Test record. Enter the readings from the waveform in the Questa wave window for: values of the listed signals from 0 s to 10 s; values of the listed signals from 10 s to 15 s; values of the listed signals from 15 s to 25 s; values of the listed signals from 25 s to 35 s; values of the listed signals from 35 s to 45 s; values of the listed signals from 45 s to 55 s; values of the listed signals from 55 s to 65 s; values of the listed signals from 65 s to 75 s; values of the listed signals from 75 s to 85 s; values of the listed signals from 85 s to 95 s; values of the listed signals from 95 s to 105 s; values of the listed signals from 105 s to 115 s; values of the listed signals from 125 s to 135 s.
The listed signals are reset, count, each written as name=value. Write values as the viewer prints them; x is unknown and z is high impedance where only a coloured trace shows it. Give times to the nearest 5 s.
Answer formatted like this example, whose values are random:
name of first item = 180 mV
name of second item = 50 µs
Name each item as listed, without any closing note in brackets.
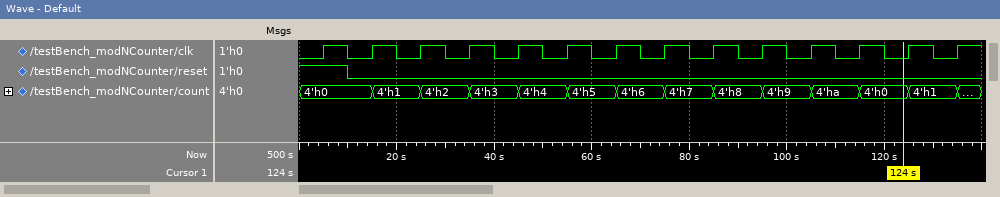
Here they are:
values of the listed signals from 0 s to 10 s = reset=1, count=4'h0
values of the listed signals from 10 s to 15 s = reset=0, count=4'h0
values of the listed signals from 15 s to 25 s = reset=0, count=4'h1
values of the listed signals from 25 s to 35 s = reset=0, count=4'h2
values of the listed signals from 35 s to 45 s = reset=0, count=4'h3
values of the listed signals from 45 s to 55 s = reset=0, count=4'h4
values of the listed signals from 55 s to 65 s = reset=0, count=4'h5
values of the listed signals from 65 s to 75 s = reset=0, count=4'h6
values of the listed signals from 75 s to 85 s = reset=0, count=4'h7
values of the listed signals from 85 s to 95 s = reset=0, count=4'h8
values of the listed signals from 95 s to 105 s = reset=0, count=4'h9
values of the listed signals from 105 s to 115 s = reset=0, count=4'ha
values of the listed signals from 125 s to 135 s = reset=0, count=4'h1
